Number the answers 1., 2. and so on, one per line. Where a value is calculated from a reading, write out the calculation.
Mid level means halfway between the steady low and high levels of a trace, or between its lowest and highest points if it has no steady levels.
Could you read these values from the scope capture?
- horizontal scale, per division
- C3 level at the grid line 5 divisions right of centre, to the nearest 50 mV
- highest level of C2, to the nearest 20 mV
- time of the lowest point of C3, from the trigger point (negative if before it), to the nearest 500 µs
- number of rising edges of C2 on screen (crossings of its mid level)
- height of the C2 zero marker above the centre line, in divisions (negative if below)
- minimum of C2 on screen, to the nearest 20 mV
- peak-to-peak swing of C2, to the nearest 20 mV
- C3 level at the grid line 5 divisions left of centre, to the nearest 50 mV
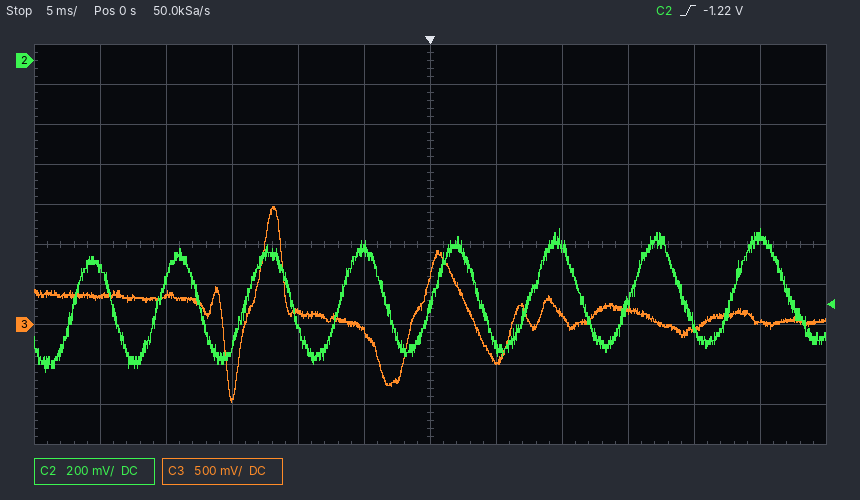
1. 5 ms
2. 50 mV
3. -840 mV
4. -15.0 ms
5. 8
6. +4.6 div
7. -1.56 V
8. -840 mV − (-1.56 V) = 720 mV
9. 350 mV
